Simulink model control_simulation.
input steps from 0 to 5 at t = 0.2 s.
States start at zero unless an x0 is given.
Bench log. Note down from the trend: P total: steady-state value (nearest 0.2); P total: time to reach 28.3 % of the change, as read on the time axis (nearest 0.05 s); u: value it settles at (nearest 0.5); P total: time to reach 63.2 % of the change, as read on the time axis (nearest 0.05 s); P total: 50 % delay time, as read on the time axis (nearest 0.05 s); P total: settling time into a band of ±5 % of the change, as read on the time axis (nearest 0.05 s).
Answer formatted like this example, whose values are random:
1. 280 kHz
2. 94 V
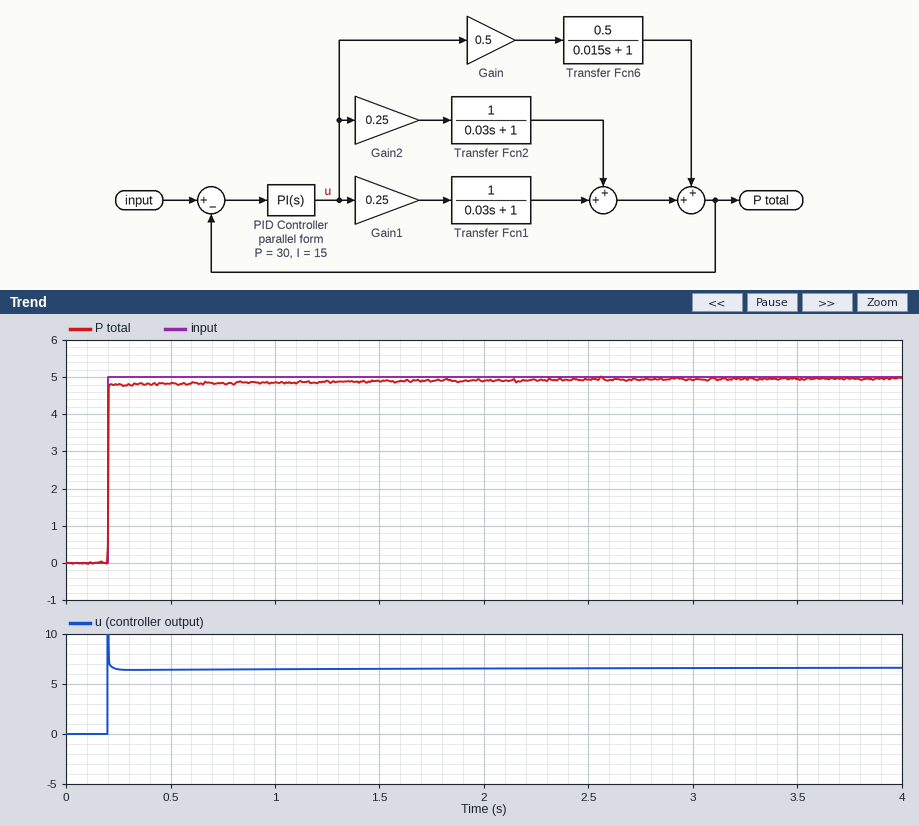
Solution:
1. 5.0
2. 0.20 s
3. 6.5
4. 0.20 s
5. 0.20 s
6. 0.20 s
